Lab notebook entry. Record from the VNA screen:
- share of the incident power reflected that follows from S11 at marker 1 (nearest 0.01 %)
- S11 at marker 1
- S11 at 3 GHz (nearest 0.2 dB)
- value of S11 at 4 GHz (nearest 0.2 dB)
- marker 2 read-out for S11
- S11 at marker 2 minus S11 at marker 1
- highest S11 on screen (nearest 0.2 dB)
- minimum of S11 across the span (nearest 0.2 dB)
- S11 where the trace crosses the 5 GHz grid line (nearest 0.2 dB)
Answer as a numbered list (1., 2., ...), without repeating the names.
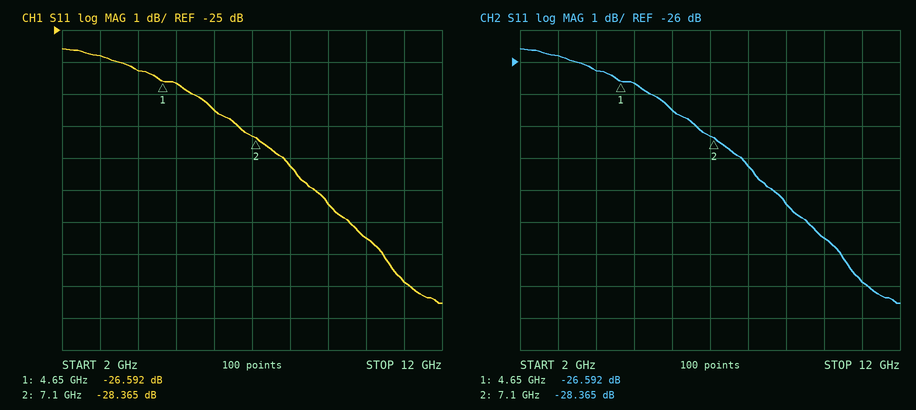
1. 0.22 %
2. -26.592 dB
3. -25.8 dB
4. -26.2 dB
5. -28.365 dB
6. -1.773 dB
7. -25.6 dB
8. -33.6 dB
9. -26.6 dB
